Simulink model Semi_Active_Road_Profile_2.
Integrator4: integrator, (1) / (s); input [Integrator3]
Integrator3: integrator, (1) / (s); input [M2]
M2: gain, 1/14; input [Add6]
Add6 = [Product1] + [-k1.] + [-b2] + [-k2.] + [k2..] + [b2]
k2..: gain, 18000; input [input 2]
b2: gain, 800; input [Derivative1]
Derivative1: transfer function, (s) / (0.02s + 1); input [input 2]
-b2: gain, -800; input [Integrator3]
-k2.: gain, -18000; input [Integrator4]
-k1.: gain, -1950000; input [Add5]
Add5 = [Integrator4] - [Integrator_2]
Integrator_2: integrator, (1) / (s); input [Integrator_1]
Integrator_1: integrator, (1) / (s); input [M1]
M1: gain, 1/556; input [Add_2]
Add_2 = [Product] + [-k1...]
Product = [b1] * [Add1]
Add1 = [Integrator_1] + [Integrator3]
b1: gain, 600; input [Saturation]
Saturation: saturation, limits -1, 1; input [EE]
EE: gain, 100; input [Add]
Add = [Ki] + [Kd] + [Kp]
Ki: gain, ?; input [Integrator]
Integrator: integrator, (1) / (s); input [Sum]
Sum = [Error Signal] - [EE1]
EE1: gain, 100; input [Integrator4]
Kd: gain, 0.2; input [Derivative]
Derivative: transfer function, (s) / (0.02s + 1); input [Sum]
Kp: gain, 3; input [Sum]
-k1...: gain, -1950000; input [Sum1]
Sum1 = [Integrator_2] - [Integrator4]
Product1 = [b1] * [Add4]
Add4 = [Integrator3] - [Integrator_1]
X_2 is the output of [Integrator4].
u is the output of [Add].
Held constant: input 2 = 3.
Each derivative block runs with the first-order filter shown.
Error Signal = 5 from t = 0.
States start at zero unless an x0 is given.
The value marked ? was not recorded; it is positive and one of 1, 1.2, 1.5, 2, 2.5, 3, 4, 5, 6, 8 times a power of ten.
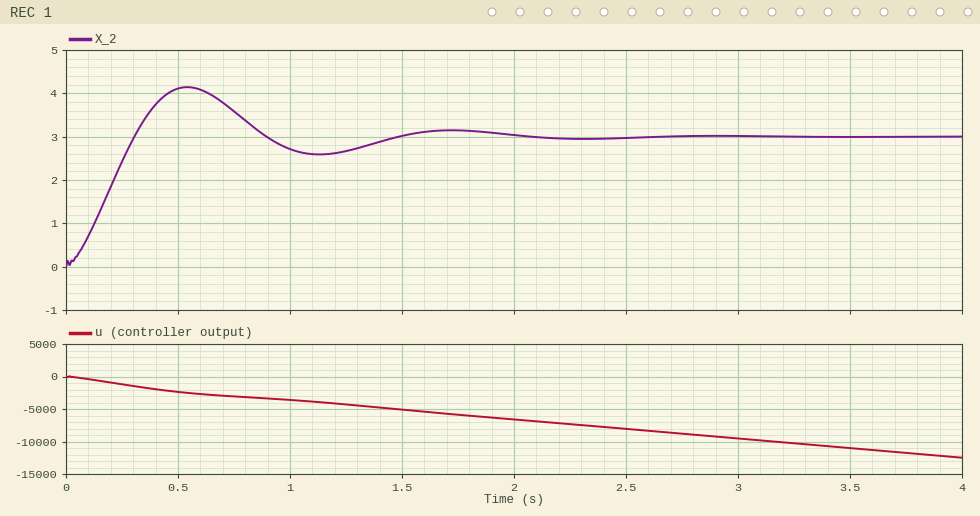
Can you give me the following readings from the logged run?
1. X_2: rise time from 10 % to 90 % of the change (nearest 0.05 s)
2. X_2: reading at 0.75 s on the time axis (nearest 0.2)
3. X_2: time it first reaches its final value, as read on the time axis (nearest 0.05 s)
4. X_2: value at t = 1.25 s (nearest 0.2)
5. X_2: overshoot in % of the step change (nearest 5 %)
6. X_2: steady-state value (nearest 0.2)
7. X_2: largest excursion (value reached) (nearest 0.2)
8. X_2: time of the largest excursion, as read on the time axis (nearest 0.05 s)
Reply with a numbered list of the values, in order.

1. 0.20 s
2. 3.6
3. 0.30 s
4. 2.6
5. 40 %
6. 3.0
7. 4.2
8. 0.55 s
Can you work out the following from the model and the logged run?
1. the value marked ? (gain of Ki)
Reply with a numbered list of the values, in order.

1. 10
